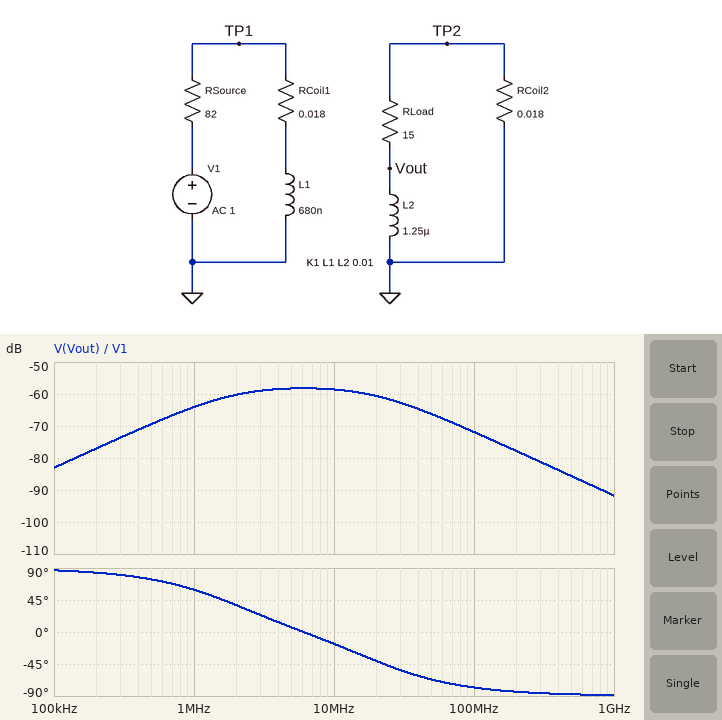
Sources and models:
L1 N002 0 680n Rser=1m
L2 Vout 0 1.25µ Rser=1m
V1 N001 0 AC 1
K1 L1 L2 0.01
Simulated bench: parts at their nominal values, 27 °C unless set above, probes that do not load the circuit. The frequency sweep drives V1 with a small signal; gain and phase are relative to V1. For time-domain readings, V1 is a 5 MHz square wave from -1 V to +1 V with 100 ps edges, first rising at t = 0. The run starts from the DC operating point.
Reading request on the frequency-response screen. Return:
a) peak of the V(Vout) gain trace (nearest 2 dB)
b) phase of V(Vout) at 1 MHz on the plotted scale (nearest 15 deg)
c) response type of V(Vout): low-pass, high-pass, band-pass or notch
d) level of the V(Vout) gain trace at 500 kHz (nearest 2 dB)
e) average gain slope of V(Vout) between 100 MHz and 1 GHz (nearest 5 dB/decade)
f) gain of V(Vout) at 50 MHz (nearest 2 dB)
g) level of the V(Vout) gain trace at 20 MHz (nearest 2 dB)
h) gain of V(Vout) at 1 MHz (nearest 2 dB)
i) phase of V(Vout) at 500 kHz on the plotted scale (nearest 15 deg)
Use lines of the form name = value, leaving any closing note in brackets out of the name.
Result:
peak of the V(Vout) gain trace = -58 dB
phase of V(Vout) at 1 MHz on the plotted scale = 60 deg
response type of V(Vout): low-pass, high-pass, band-pass or notch = band-pass
level of the V(Vout) gain trace at 500 kHz = -70 dB
average gain slope of V(Vout) between 100 MHz and 1 GHz = -20 dB/decade
gain of V(Vout) at 50 MHz = -66 dB
level of the V(Vout) gain trace at 20 MHz = -60 dB
gain of V(Vout) at 1 MHz = -64 dB
phase of V(Vout) at 500 kHz on the plotted scale = 75 deg
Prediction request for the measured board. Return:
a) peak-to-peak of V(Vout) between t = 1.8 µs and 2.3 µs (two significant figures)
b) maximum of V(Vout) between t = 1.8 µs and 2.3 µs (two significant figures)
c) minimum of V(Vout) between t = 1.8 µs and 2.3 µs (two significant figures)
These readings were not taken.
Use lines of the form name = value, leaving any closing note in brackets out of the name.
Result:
peak-to-peak of V(Vout) between t = 1.8 µs and 2.3 µs = 3.1 mV
maximum of V(Vout) between t = 1.8 µs and 2.3 µs = 1.6 mV
minimum of V(Vout) between t = 1.8 µs and 2.3 µs = -1.6 mV
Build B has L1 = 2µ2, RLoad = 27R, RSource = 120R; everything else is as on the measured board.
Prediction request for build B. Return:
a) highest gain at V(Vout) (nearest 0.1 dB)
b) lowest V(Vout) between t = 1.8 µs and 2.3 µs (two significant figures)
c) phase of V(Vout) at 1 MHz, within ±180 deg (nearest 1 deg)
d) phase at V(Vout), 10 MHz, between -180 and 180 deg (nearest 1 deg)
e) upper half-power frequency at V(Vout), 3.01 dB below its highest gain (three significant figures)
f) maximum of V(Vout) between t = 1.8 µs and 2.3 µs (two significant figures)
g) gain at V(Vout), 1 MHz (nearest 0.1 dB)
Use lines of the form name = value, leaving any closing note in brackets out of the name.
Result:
highest gain at V(Vout) = -53.4 dB
lowest V(Vout) between t = 1.8 µs and 2.3 µs = -2.7 mV
phase of V(Vout) at 1 MHz, within ±180 deg = 67 deg
phase at V(Vout), 10 MHz, between -180 and 180 deg = -30 deg
upper half-power frequency at V(Vout), 3.01 dB below its highest gain = 14.2 MHz
maximum of V(Vout) between t = 1.8 µs and 2.3 µs = 2.7 mV
gain at V(Vout), 1 MHz = -61.6 dB
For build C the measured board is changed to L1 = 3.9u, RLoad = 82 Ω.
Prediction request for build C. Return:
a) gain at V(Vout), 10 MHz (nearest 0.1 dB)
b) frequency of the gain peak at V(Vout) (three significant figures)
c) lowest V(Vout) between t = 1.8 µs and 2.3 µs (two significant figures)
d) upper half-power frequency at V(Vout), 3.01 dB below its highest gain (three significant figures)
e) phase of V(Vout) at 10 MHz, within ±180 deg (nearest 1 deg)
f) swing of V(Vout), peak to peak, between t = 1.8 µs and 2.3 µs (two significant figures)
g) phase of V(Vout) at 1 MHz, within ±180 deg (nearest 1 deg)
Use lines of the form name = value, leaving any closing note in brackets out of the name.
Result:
gain at V(Vout), 10 MHz = -48.2 dB
frequency of the gain peak at V(Vout) = 5.91 MHz
lowest V(Vout) between t = 1.8 µs and 2.3 µs = -5.6 mV
upper half-power frequency at V(Vout), 3.01 dB below its highest gain = 16.0 MHz
phase of V(Vout) at 10 MHz, within ±180 deg = -25 deg
swing of V(Vout), peak to peak, between t = 1.8 µs and 2.3 µs = 11 mV
phase of V(Vout) at 1 MHz, within ±180 deg = 68 deg
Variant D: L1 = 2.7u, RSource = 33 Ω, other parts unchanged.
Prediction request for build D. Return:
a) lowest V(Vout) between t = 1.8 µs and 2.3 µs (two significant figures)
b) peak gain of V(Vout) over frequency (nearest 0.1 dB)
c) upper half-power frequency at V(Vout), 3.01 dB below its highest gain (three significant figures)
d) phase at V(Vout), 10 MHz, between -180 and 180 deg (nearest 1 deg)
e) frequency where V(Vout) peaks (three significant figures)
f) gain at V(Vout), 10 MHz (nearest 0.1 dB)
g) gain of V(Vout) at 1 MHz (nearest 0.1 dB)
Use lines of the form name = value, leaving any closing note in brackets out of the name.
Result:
lowest V(Vout) between t = 1.8 µs and 2.3 µs = -2.9 mV
peak gain of V(Vout) over frequency = -49.4 dB
upper half-power frequency at V(Vout), 3.01 dB below its highest gain = 4.66 MHz
phase at V(Vout), 10 MHz, between -180 and 180 deg = -68 deg
frequency where V(Vout) peaks = 1.93 MHz
gain at V(Vout), 10 MHz = -58.0 dB
gain of V(Vout) at 1 MHz = -51.2 dB
